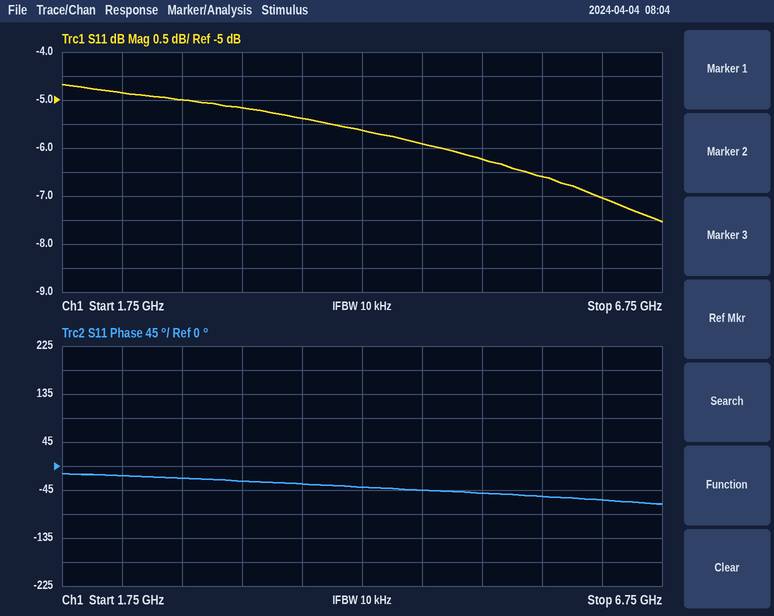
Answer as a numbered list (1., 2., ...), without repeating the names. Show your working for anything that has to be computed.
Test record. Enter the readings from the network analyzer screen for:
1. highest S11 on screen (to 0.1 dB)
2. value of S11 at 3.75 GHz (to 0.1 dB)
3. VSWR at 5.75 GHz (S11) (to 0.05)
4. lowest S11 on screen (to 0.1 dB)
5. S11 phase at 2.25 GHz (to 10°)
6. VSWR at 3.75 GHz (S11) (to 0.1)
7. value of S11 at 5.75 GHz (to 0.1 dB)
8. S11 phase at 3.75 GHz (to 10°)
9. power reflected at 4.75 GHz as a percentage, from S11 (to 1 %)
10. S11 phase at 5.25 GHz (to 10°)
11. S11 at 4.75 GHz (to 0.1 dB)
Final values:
1. -4.7 dB
2. -5.4 dB
3. |Γ| = 10^(-6.6/20) = 0.4677; VSWR = (1 + 0.4677)/(1 − 0.4677) ≈ 2.76, so 2.75 to the nearest 0.05
4. -7.5 dB
5. -20°
6. |Γ| = 10^(-5.4/20) = 0.5370; VSWR = (1 + 0.5370)/(1 − 0.5370) ≈ 3.3
7. -6.6 dB
8. -30°
9. 10^(-5.9/10) ≈ 26 %
10. -50°
11. -5.9 dB
